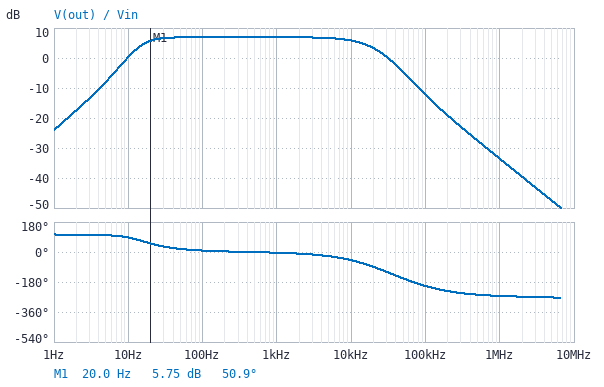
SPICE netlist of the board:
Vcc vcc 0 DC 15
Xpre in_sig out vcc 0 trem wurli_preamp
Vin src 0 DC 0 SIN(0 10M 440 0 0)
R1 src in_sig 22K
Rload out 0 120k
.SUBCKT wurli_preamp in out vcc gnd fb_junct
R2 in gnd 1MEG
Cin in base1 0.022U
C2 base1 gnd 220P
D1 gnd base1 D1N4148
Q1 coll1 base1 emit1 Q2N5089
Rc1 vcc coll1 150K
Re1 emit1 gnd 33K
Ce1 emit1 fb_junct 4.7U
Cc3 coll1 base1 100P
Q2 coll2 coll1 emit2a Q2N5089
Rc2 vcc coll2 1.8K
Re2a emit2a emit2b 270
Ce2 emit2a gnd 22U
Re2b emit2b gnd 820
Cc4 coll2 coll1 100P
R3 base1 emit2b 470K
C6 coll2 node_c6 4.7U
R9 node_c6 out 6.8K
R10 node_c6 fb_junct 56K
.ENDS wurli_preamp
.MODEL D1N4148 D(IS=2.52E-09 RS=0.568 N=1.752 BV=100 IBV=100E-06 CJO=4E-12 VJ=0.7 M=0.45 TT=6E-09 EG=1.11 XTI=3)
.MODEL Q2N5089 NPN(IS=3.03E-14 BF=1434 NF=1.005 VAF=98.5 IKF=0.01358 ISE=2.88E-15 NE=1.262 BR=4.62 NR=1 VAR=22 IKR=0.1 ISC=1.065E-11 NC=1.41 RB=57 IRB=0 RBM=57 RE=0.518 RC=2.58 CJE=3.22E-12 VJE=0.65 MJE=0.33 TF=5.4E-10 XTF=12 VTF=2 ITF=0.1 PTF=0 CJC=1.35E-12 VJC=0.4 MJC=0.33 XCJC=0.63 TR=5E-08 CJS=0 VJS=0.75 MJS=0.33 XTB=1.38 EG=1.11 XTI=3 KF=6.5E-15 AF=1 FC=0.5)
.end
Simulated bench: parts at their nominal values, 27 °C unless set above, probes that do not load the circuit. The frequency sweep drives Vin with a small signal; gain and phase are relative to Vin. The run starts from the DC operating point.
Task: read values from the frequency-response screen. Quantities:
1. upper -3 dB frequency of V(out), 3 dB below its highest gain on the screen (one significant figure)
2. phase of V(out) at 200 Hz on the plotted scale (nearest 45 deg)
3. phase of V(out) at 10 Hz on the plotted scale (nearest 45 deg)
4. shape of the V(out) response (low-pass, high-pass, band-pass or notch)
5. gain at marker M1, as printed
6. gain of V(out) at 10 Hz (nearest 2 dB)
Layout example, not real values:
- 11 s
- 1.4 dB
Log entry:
- 20 kHz
- 0 deg
- 90 deg
- band-pass
- 5.75 dB
- 0 dB
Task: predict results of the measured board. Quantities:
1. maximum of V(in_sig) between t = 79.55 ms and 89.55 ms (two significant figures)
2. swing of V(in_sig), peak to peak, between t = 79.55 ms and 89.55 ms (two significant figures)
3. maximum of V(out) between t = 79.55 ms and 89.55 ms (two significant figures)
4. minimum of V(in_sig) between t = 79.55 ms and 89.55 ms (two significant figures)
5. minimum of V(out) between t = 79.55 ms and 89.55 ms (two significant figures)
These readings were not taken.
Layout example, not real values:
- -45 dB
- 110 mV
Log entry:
- 9.4 mV
- 19 mV
- 22 mV
- -9.4 mV
- -22 mV
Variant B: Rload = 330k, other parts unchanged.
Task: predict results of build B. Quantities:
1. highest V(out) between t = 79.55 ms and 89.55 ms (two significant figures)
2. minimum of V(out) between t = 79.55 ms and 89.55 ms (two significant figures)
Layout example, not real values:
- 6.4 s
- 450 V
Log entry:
- 23 mV
- -23 mV
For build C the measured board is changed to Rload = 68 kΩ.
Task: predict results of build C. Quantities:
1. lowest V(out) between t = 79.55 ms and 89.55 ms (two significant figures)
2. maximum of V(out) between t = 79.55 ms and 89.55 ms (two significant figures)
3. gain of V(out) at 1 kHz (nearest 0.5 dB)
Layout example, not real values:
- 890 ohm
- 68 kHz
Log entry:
- -21 mV
- 21 mV
- 6.5 dB
